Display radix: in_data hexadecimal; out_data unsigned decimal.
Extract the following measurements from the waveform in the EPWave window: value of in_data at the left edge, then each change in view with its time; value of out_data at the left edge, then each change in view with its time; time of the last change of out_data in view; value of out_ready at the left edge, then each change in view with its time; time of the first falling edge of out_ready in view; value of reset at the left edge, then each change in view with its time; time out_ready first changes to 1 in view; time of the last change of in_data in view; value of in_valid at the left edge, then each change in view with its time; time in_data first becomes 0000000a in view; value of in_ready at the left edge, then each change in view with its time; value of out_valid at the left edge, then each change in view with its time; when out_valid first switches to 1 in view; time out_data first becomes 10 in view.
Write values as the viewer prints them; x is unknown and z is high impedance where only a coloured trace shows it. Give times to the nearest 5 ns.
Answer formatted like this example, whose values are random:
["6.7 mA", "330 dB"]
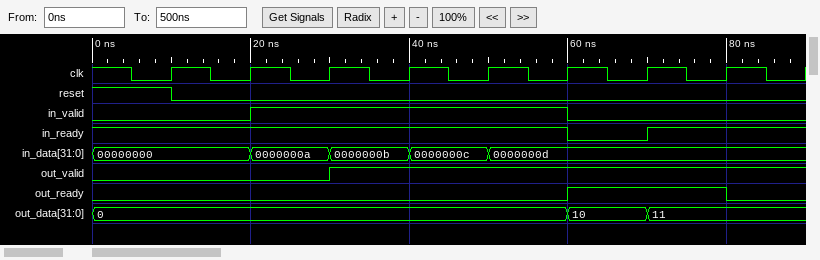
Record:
["00000000, 0000000a at 20 ns, 0000000b at 30 ns, 0000000c at 40 ns, 0000000d at 50 ns", "0, 10 at 60 ns, 11 at 70 ns", "70 ns", "0, 1 at 60 ns, 0 at 80 ns", "80 ns", "1, 0 at 10 ns", "60 ns", "50 ns", "0, 1 at 20 ns, 0 at 60 ns", "20 ns", "1, 0 at 60 ns, 1 at 70 ns", "0, 1 at 30 ns", "30 ns", "60 ns"]
